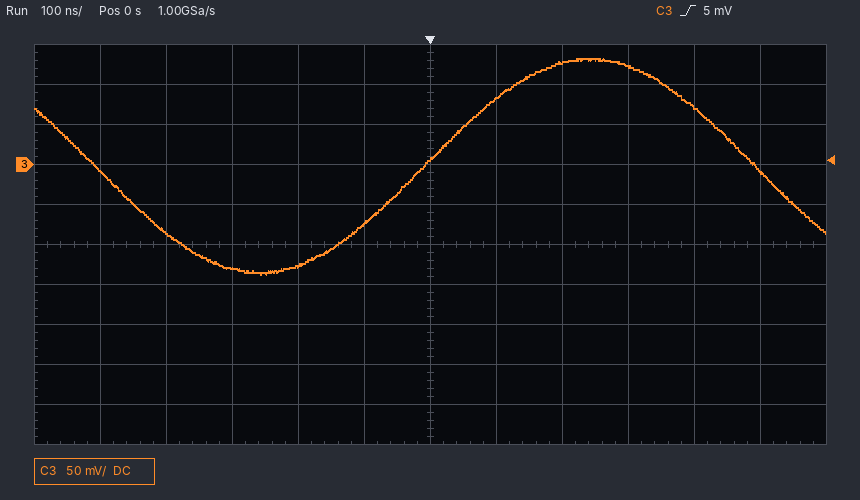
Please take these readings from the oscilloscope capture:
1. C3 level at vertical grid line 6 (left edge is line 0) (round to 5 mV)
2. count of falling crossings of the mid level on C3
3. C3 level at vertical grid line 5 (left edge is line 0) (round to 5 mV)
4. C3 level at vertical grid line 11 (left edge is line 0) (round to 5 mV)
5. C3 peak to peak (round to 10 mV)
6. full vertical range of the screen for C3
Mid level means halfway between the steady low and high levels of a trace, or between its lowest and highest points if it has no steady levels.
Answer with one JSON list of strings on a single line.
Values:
["5 mV", "2", "-75 mV", "-10 mV", "270 mV", "500 mV"]
